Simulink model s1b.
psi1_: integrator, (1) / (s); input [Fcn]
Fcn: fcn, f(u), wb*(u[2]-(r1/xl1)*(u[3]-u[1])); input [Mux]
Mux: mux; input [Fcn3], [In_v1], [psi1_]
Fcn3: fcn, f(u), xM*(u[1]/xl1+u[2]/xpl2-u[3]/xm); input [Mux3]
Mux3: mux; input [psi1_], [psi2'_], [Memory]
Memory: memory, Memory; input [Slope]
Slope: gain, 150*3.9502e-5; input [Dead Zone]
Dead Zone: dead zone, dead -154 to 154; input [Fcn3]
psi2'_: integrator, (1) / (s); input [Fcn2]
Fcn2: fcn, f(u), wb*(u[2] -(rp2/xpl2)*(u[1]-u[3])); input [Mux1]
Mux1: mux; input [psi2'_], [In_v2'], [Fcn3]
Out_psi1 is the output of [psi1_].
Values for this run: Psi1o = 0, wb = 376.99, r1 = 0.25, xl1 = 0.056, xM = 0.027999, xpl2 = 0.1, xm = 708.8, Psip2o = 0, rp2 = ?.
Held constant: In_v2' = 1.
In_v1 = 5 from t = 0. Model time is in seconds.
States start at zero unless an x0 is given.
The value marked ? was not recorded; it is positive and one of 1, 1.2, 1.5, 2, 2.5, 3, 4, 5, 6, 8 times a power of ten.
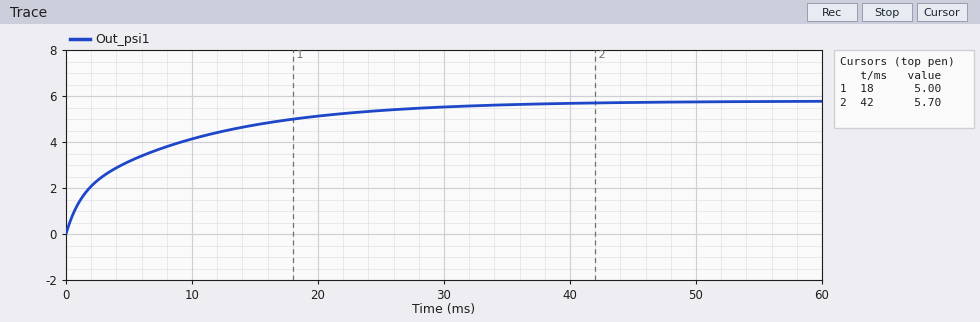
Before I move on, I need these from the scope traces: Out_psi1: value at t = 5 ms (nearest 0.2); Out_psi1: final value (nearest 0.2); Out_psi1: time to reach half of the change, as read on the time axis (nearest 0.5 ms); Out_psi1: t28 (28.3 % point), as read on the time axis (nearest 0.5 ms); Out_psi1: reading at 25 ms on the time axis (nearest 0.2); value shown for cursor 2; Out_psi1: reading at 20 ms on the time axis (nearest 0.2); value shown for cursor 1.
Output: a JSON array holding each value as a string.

["3.2", "5.8", "4.0 ms", "1.5 ms", "5.4", "5.70", "5.2", "5.00"]
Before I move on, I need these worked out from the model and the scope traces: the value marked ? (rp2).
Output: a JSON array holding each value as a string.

["0.06"]
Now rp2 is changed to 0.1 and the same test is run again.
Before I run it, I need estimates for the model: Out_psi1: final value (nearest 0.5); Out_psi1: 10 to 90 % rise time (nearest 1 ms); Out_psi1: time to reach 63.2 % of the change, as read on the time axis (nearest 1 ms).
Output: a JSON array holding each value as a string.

["5.0", "13 ms", "5 ms"]
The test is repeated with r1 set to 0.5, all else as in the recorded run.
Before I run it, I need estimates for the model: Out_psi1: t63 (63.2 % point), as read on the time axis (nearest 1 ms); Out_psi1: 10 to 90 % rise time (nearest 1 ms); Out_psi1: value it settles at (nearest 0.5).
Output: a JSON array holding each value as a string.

["8 ms", "21 ms", "4.0"]
